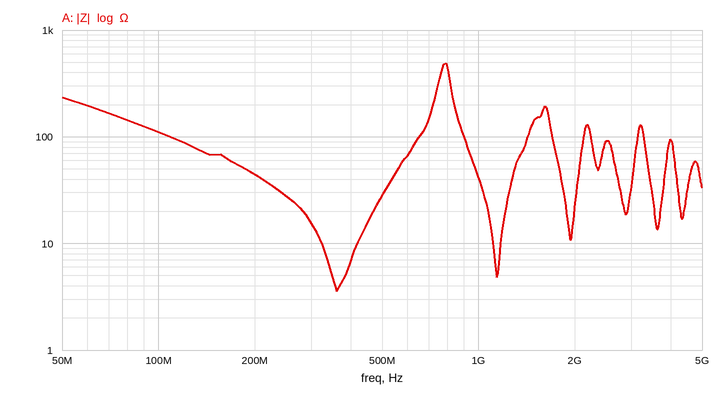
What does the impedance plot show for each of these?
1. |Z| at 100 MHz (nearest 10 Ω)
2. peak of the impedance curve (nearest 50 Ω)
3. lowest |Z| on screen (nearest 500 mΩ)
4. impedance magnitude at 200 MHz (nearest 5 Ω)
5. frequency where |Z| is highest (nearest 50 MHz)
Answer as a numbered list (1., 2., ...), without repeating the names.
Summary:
1. 110 Ω
2. 500 Ω
3. 3.5 Ω
4. 45 Ω
5. 800 MHz
